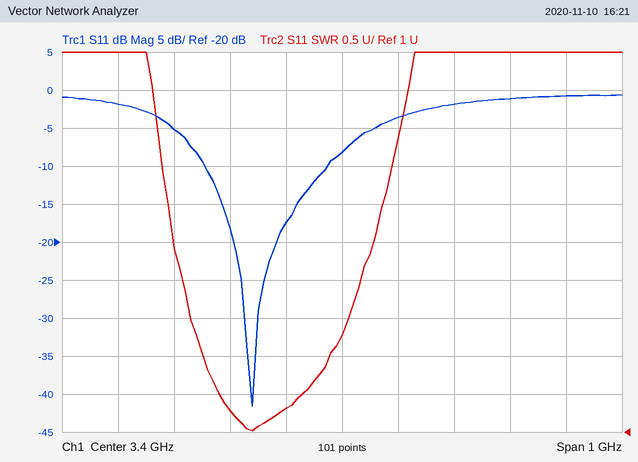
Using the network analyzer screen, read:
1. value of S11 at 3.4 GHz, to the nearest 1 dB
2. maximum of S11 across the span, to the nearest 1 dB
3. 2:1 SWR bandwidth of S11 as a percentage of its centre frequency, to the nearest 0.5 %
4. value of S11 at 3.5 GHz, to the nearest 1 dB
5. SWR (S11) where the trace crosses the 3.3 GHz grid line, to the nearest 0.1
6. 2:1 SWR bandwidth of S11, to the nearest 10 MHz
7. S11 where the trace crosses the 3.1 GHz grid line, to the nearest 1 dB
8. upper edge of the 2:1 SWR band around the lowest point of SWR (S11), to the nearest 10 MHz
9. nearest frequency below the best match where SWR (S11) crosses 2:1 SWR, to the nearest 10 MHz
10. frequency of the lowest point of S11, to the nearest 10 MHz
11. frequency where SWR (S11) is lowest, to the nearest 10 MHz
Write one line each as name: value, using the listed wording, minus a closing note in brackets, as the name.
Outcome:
value of S11 at 3.4 GHz, to the nearest 1 dB: -8 dB
maximum of S11 across the span, to the nearest 1 dB: -1 dB
2:1 SWR bandwidth of S11 as a percentage of its centre frequency, to the nearest 0.5 %: 7.0 %
value of S11 at 3.5 GHz, to the nearest 1 dB: -4 dB
SWR (S11) where the trace crosses the 3.3 GHz grid line, to the nearest 0.1: 1.3
2:1 SWR bandwidth of S11, to the nearest 10 MHz: 230 MHz
S11 where the trace crosses the 3.1 GHz grid line, to the nearest 1 dB: -5 dB
upper edge of the 2:1 SWR band around the lowest point of SWR (S11), to the nearest 10 MHz: 3.38 GHz
nearest frequency below the best match where SWR (S11) crosses 2:1 SWR, to the nearest 10 MHz: 3.15 GHz
frequency of the lowest point of S11, to the nearest 10 MHz: 3.24 GHz
frequency where SWR (S11) is lowest, to the nearest 10 MHz: 3.24 GHz
